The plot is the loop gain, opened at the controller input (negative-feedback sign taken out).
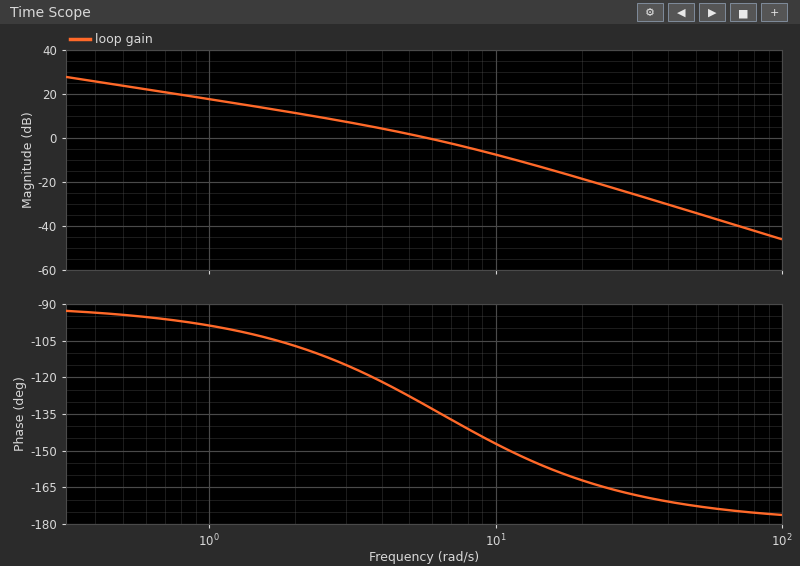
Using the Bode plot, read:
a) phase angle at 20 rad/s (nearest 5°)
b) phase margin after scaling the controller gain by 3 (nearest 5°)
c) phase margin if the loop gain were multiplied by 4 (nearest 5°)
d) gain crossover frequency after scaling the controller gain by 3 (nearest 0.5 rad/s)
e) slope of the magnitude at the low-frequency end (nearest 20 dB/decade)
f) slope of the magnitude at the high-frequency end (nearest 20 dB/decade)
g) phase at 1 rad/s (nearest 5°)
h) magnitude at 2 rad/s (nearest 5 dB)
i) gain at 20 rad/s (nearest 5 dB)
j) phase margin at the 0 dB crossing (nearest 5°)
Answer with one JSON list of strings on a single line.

["-160°", "30°", "25°", "11.5 rad/s", "-20 dB/decade", "-40 dB/decade", "-100°", "10 dB", "-20 dB", "50°"]
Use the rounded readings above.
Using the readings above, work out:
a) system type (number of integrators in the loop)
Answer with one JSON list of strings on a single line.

["1"]
